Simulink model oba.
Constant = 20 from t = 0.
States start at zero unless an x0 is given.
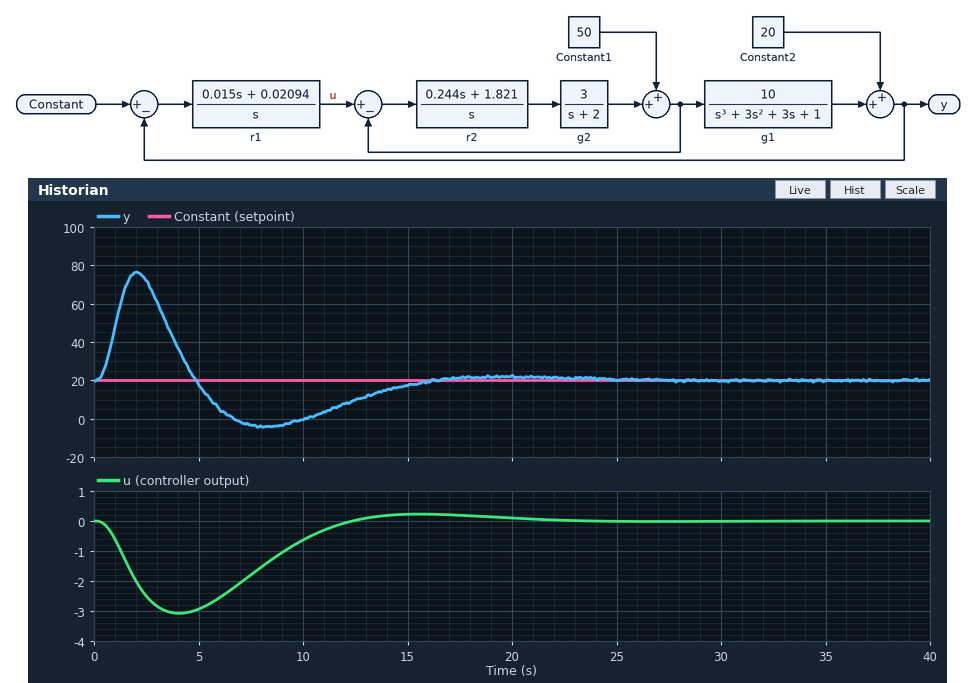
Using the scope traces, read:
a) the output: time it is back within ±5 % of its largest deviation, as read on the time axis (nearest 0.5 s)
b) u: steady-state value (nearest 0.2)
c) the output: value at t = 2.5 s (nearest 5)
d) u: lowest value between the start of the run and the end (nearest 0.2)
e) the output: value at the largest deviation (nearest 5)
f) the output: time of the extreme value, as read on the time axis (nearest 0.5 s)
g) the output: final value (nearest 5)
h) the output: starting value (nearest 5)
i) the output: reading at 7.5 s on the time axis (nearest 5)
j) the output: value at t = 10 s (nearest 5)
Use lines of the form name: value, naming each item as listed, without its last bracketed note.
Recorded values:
the output: time it is back within ±5 % of its largest deviation, as read on the time axis: 15.0 s
u: steady-state value: 0.0
the output: value at t = 2.5 s: 70
u: lowest value between the start of the run and the end: -3.0
the output: value at the largest deviation: 75
the output: time of the extreme value, as read on the time axis: 2.0 s
the output: final value: 20
the output: starting value: 20
the output: reading at 7.5 s on the time axis: -5
the output: value at t = 10 s: 0
